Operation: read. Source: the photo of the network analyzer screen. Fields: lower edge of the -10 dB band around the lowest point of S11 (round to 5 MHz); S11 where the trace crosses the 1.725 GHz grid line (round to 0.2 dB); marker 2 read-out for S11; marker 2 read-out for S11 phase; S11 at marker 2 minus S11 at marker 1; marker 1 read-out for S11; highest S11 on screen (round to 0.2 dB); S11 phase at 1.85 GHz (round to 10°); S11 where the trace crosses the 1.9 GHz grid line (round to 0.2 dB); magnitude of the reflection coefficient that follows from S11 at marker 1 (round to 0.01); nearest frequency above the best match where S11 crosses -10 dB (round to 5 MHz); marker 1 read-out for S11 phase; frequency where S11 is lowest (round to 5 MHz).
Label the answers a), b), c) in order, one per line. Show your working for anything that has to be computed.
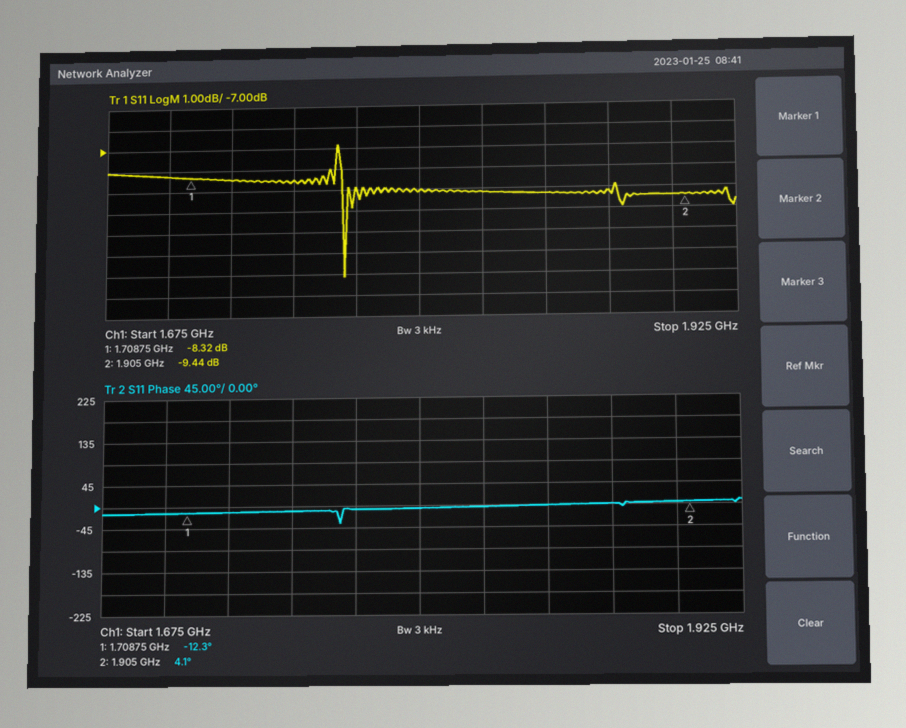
a) 1.770 GHz
b) -8.4 dB
c) -9.44 dB
d) 4.1°
e) -9.44 − (-8.32) = -1.12 dB
f) -8.32 dB
g) -6.8 dB
h) 0°
i) -9.4 dB
j) 10^(-8.32/20) ≈ 0.38
k) 1.770 GHz
l) -12.3°
m) 1.770 GHz
